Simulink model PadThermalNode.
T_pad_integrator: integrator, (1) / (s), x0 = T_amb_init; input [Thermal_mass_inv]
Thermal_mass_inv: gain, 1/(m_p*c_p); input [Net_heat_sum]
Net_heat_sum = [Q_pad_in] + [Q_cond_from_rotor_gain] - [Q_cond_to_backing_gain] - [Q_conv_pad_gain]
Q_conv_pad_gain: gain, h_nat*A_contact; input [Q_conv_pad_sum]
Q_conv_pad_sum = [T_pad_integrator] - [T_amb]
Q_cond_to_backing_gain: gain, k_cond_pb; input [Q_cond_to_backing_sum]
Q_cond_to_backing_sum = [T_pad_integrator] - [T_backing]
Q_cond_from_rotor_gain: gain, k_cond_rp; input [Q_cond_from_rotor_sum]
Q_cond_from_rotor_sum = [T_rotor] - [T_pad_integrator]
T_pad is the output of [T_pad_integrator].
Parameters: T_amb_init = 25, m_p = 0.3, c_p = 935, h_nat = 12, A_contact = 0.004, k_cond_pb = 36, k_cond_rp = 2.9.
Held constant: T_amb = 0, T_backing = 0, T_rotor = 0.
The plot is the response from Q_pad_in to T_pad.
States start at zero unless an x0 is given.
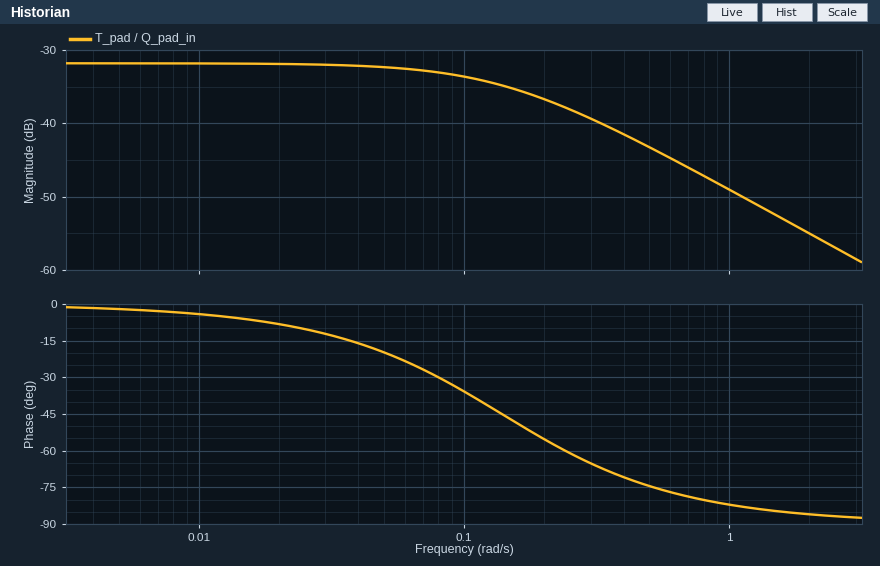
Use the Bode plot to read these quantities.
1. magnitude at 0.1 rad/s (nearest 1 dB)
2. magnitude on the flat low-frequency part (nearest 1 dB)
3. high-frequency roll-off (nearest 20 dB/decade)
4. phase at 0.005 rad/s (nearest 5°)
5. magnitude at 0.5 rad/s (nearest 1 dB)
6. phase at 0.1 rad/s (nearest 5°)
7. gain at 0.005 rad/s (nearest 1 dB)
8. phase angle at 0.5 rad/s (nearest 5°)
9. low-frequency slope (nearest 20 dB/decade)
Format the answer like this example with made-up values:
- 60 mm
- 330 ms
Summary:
- -34 dB
- -32 dB
- -20 dB/decade
- 0°
- -43 dB
- -35°
- -32 dB
- -75°
- 0 dB/decade
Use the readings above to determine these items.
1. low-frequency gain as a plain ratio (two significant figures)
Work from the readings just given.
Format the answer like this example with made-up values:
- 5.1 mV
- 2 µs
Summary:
- 0.025
